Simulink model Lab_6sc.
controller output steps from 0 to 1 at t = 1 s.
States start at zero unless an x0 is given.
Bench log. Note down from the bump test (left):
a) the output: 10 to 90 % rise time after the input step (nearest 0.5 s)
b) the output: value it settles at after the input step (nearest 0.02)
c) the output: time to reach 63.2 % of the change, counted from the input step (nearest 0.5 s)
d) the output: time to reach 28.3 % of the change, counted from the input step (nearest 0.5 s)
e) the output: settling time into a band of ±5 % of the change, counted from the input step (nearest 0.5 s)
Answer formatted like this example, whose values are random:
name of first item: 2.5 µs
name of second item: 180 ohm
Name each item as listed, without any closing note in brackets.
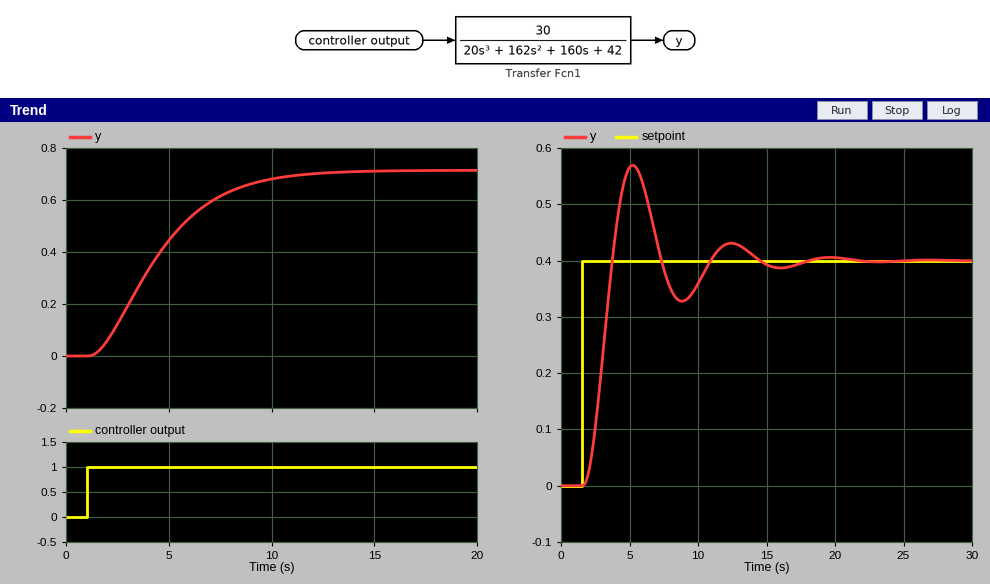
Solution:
the output: 10 to 90 % rise time after the input step: 6.0 s
the output: value it settles at after the input step: 0.72
the output: time to reach 63.2 % of the change, counted from the input step: 4.0 s
the output: time to reach 28.3 % of the change, counted from the input step: 2.0 s
the output: settling time into a band of ±5 % of the change, counted from the input step: 9.0 s
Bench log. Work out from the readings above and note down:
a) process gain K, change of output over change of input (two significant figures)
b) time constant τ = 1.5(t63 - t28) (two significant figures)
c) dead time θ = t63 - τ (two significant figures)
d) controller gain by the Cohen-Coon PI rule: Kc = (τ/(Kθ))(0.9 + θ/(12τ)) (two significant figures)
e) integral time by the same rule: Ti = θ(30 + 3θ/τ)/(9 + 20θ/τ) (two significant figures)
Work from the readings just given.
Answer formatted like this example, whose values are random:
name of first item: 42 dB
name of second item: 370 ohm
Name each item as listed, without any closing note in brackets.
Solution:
process gain K, change of output over change of input: 0.72
time constant τ = 1.5(t63 - t28): 3.0 s
dead time θ = t63 - τ: 1.0 s
controller gain by the Cohen-Coon PI rule: Kc = (τ/(Kθ))(0.9 + θ/(12τ)): 3.9
integral time by the same rule: Ti = θ(30 + 3θ/τ)/(9 + 20θ/τ): 2.0 s
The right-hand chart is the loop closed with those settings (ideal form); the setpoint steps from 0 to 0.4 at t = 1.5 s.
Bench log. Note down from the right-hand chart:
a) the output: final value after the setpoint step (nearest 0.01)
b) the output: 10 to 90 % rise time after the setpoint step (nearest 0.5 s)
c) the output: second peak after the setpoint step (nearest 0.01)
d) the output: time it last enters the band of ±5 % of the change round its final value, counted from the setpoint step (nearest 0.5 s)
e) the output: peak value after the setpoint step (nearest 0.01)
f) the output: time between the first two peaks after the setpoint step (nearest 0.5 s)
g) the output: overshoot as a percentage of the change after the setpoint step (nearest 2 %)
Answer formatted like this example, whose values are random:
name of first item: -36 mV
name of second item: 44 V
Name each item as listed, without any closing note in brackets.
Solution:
the output: final value after the setpoint step: 0.40
the output: 10 to 90 % rise time after the setpoint step: 1.5 s
the output: second peak after the setpoint step: 0.43
the output: time it last enters the band of ±5 % of the change round its final value, counted from the setpoint step: 12.0 s
the output: peak value after the setpoint step: 0.57
the output: time between the first two peaks after the setpoint step: 7.0 s
the output: overshoot as a percentage of the change after the setpoint step: 42 %
